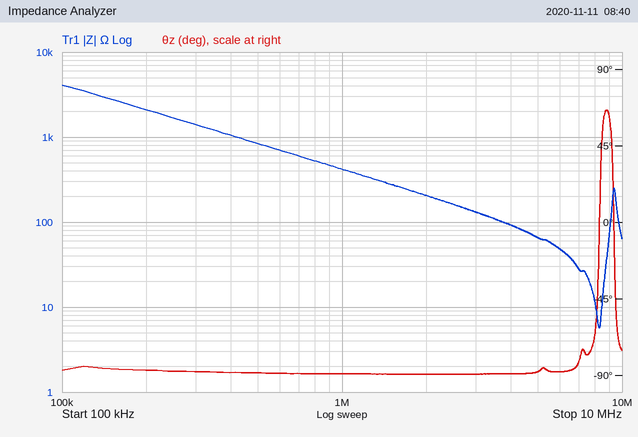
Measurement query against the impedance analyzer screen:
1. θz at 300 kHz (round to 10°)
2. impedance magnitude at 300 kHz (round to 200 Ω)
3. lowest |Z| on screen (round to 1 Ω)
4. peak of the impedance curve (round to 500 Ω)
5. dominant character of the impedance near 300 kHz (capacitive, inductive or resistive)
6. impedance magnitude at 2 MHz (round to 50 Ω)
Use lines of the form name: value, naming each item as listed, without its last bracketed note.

θz at 300 kHz: -90°
impedance magnitude at 300 kHz: 1.4 kΩ
lowest |Z| on screen: 6 Ω
peak of the impedance curve: 4.0 kΩ
dominant character of the impedance near 300 kHz: capacitive
impedance magnitude at 2 MHz: 200 Ω
